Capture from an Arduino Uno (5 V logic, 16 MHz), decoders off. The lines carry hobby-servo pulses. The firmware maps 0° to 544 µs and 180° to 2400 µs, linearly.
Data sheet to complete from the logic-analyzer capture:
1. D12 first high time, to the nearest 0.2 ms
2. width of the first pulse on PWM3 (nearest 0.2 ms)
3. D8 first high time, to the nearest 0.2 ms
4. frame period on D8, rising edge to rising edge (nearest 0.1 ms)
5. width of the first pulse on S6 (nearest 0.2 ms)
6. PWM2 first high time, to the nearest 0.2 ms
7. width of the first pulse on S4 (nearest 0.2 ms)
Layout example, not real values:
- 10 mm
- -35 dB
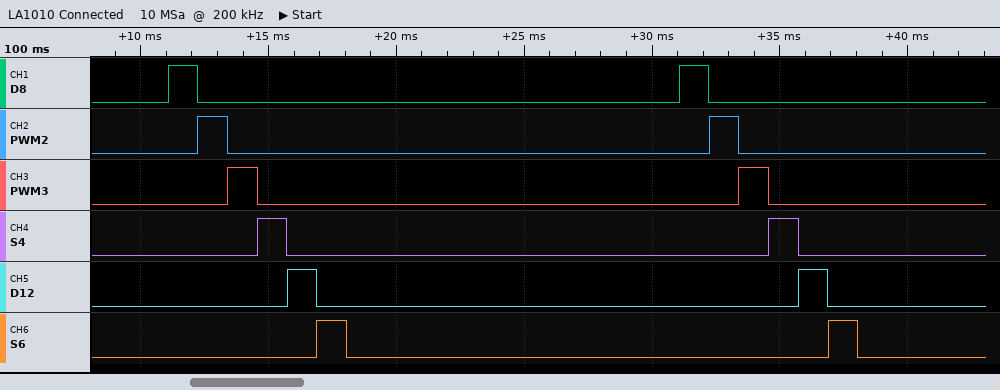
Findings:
- 1.2 ms
- 1.2 ms
- 1.2 ms
- 20.0 ms
- 1.2 ms
- 1.2 ms
- 1.2 ms
